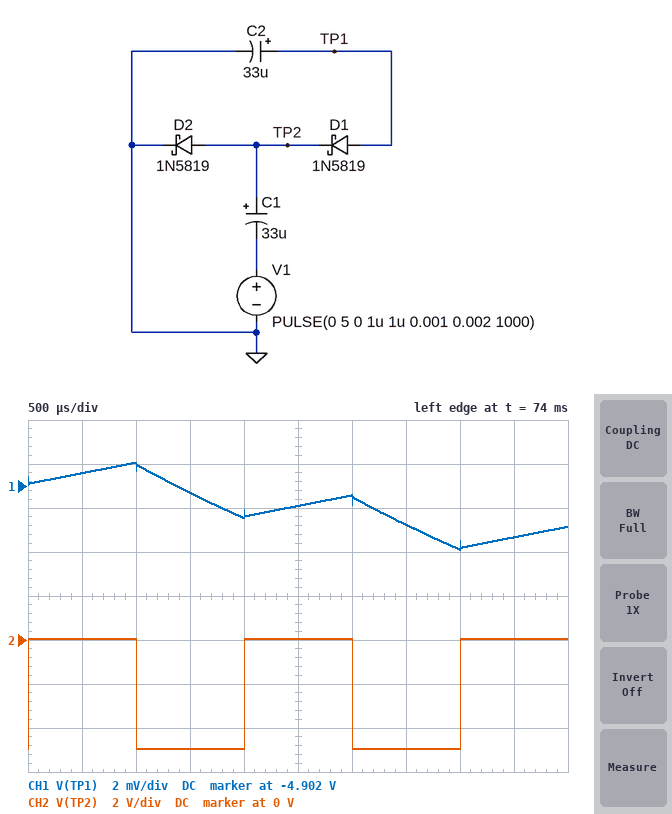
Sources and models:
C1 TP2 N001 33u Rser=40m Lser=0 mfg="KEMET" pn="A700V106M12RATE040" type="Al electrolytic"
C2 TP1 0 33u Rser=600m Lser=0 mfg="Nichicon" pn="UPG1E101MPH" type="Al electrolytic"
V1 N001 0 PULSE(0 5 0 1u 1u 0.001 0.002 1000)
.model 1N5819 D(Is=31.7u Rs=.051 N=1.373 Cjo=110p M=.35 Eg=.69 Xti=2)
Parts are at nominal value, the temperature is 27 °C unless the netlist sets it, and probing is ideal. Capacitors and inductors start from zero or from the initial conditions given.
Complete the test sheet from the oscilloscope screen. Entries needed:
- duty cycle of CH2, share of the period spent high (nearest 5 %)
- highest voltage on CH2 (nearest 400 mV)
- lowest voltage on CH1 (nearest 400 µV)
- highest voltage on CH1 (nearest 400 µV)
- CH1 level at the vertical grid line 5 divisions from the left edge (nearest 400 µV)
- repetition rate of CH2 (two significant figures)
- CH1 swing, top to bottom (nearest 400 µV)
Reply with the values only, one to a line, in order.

50 %
0 V
-4.9048 V
-4.9008 V
-4.9028 V
500 Hz
4.0 mV
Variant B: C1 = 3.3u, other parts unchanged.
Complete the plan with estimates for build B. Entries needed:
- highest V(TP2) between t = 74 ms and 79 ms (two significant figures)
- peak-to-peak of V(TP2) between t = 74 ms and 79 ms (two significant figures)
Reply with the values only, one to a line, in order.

210 mV
5.2 V
